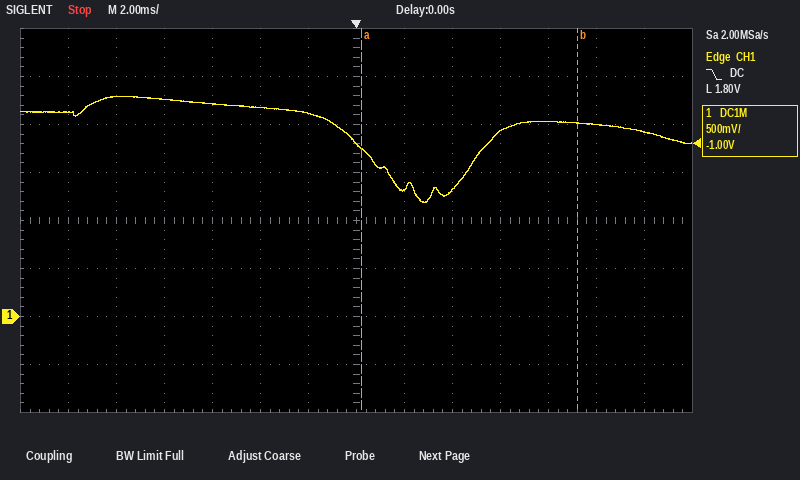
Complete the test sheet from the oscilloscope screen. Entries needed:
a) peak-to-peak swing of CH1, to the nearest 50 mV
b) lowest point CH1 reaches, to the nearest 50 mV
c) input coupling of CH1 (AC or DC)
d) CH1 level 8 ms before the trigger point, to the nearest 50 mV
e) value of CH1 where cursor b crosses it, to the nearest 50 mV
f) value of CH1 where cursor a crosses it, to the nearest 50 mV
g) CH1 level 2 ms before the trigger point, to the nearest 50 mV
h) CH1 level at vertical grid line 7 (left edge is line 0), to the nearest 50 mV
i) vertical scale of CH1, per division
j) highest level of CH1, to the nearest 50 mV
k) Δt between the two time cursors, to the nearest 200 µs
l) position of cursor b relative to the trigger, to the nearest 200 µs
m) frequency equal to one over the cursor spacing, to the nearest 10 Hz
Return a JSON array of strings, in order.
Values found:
["1.10 V", "1.20 V", "DC", "2.25 V", "2.00 V", "1.75 V", "2.10 V", "1.80 V", "500 mV", "2.30 V", "9.0 ms", "+9.2 ms", "110 Hz"]
